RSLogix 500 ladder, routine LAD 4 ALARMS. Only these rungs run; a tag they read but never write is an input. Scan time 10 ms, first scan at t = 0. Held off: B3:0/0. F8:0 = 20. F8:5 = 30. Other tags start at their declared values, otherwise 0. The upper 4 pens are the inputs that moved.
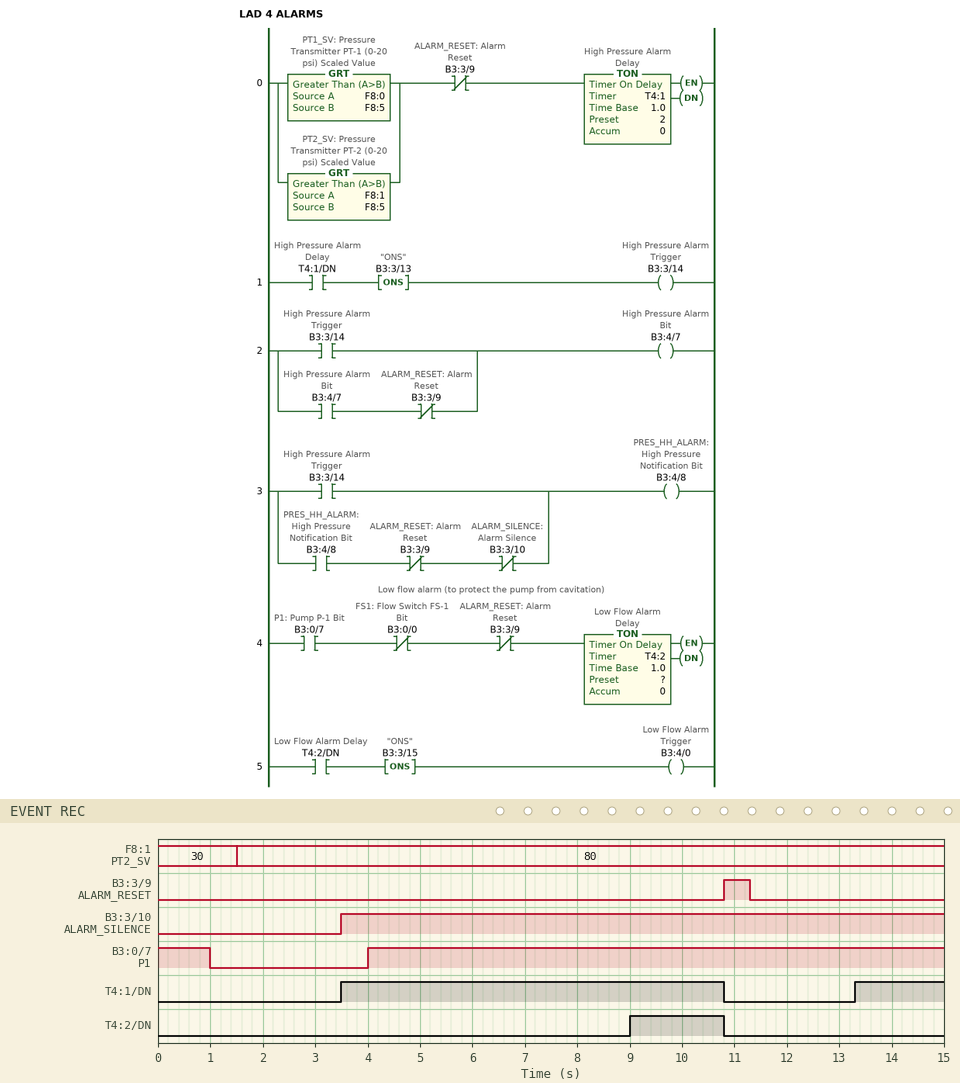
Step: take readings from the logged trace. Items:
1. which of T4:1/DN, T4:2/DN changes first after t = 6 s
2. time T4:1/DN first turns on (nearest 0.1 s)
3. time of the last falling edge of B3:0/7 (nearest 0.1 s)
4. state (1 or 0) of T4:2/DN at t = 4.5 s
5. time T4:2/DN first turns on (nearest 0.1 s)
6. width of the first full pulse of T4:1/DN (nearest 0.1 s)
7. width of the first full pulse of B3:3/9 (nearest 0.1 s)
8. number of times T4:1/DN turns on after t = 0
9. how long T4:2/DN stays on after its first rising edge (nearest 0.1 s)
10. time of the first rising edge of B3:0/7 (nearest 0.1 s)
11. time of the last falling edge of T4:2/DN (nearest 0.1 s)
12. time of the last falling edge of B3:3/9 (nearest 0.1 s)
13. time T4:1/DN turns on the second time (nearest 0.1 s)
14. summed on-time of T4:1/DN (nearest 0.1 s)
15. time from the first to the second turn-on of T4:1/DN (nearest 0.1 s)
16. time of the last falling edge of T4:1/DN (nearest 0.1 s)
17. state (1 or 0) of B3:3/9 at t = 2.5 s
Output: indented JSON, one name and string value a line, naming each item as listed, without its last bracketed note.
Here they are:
{
  "which of T4:1/DN, T4:2/DN changes first after t = 6 s": "T4:2/DN",
  "time T4:1/DN first turns on": "3.5 s",
  "time of the last falling edge of B3:0/7": "1.0 s",
  "state (1 or 0) of T4:2/DN at t = 4.5 s": "0",
  "time T4:2/DN first turns on": "9.0 s",
  "width of the first full pulse of T4:1/DN": "7.3 s",
  "width of the first full pulse of B3:3/9": "0.5 s",
  "number of times T4:1/DN turns on after t = 0": "2",
  "how long T4:2/DN stays on after its first rising edge": "1.8 s",
  "time of the first rising edge of B3:0/7": "4.0 s",
  "time of the last falling edge of T4:2/DN": "10.8 s",
  "time of the last falling edge of B3:3/9": "11.3 s",
  "time T4:1/DN turns on the second time": "13.3 s",
  "summed on-time of T4:1/DN": "9.0 s",
  "time from the first to the second turn-on of T4:1/DN": "9.8 s",
  "time of the last falling edge of T4:1/DN": "10.8 s",
  "state (1 or 0) of B3:3/9 at t = 2.5 s": "0"
}
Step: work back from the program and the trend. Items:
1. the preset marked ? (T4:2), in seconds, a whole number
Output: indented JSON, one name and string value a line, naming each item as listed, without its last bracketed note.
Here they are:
{
  "the preset marked ? (T4:2), in seconds, a whole number": "5 s"
}
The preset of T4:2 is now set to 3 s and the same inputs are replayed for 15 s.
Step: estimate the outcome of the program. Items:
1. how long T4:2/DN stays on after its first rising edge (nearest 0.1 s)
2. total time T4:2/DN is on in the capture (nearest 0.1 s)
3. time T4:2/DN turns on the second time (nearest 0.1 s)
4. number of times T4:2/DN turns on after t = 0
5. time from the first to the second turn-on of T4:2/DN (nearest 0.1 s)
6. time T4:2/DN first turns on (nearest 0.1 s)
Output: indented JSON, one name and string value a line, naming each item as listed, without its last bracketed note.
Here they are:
{
  "how long T4:2/DN stays on after its first rising edge": "3.8 s",
  "total time T4:2/DN is on in the capture": "4.5 s",
  "time T4:2/DN turns on the second time": "14.3 s",
  "number of times T4:2/DN turns on after t = 0": "2",
  "time from the first to the second turn-on of T4:2/DN": "7.3 s",
  "time T4:2/DN first turns on": "7.0 s"
}
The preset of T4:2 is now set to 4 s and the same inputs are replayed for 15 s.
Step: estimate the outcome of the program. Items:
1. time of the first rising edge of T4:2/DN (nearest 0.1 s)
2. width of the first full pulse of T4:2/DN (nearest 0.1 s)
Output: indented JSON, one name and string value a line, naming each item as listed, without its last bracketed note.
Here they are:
{
  "time of the first rising edge of T4:2/DN": "8.0 s",
  "width of the first full pulse of T4:2/DN": "2.8 s"
}
